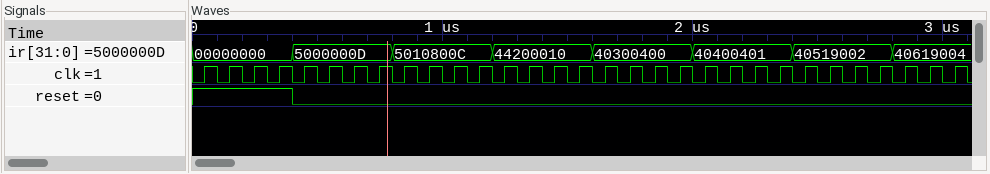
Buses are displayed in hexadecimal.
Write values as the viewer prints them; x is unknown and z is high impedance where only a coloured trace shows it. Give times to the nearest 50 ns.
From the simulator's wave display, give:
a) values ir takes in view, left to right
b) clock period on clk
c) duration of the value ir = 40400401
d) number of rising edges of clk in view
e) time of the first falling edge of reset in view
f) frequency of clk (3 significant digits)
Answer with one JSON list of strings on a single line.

["00000000, 5000000D, 5010800C, 44200010, 40300400, 40400401, 40519002, 40619004", "100 ns", "400 ns", "31", "400 ns", "10.0 MHz"]
